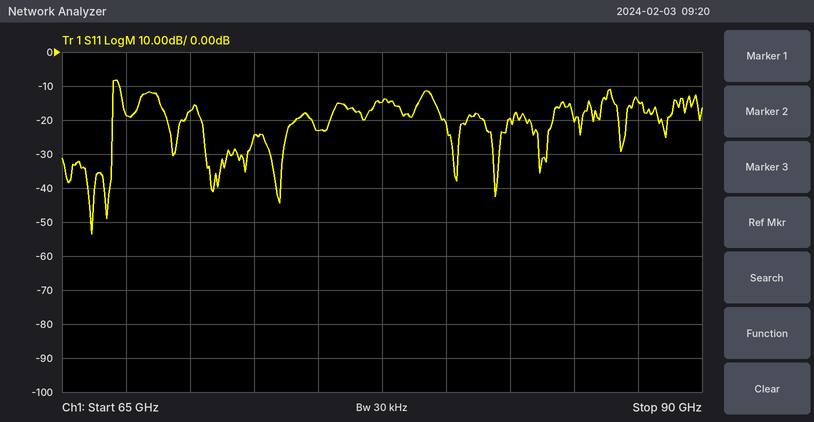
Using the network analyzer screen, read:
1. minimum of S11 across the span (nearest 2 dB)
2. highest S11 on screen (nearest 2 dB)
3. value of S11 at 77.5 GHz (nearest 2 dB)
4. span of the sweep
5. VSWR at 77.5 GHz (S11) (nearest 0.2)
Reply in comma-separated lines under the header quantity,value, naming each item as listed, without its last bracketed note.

quantity,value
minimum of S11 across the span,-54 dB
highest S11 on screen,-8 dB
value of S11 at 77.5 GHz,-14 dB
span of the sweep,25 GHz
VSWR at 77.5 GHz (S11),1.4
